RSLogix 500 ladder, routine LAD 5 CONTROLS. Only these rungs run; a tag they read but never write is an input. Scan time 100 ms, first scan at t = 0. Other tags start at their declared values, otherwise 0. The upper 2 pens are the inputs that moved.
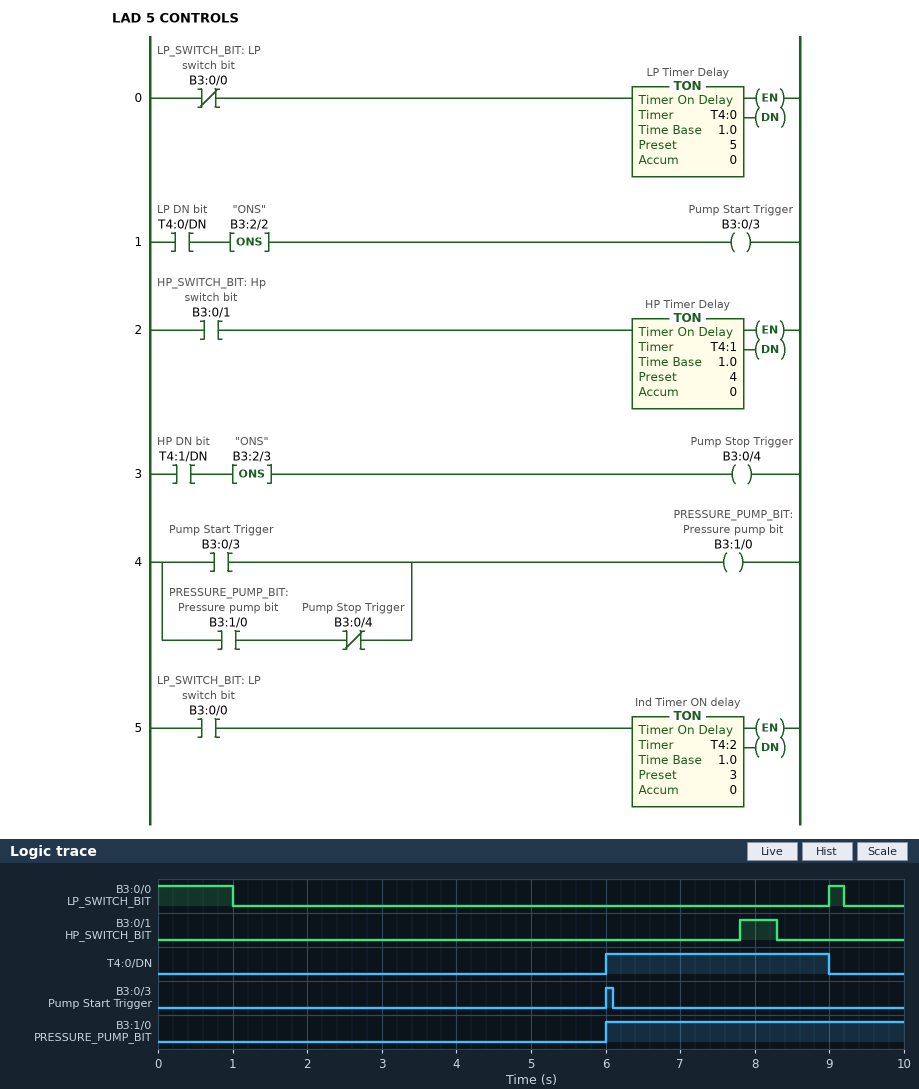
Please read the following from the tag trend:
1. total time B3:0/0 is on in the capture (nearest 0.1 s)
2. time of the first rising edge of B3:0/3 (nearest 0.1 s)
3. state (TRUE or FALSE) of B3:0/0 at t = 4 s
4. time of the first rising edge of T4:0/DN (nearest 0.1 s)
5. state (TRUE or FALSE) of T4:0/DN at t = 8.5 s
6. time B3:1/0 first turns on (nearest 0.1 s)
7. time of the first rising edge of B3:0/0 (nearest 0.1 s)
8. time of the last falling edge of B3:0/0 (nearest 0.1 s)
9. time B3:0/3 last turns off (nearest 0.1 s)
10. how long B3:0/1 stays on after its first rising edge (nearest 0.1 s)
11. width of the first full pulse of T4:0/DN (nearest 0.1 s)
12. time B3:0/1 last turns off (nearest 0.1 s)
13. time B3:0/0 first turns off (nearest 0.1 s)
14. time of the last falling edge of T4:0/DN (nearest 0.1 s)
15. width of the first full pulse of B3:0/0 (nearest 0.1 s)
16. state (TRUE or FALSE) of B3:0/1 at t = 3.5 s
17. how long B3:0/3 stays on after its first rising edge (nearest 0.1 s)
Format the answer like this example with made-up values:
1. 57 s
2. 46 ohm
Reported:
1. 1.2 s
2. 6.0 s
3. FALSE
4. 6.0 s
5. TRUE
6. 6.0 s
7. 9.0 s
8. 9.2 s
9. 6.1 s
10. 0.5 s
11. 3.0 s
12. 8.3 s
13. 1.0 s
14. 9.0 s
15. 0.2 s
16. FALSE
17. 0.1 s
